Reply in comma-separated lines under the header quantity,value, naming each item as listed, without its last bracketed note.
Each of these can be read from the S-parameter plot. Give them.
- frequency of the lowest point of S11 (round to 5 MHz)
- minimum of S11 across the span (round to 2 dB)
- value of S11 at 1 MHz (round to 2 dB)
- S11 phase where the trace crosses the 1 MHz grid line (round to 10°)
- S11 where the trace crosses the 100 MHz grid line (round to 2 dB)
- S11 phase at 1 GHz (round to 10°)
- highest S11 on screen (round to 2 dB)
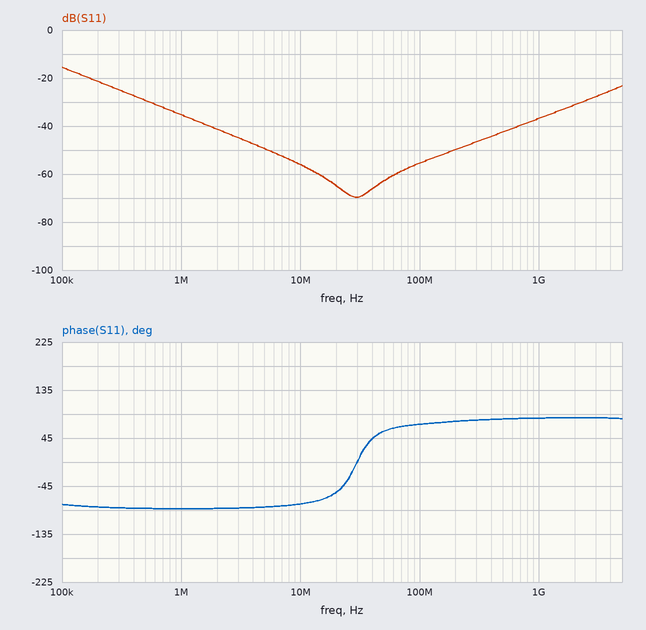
quantity,value
frequency of the lowest point of S11,30 MHz
minimum of S11 across the span,-70 dB
value of S11 at 1 MHz,-36 dB
S11 phase where the trace crosses the 1 MHz grid line,-90°
S11 where the trace crosses the 100 MHz grid line,-56 dB
S11 phase at 1 GHz,80°
highest S11 on screen,-16 dB
